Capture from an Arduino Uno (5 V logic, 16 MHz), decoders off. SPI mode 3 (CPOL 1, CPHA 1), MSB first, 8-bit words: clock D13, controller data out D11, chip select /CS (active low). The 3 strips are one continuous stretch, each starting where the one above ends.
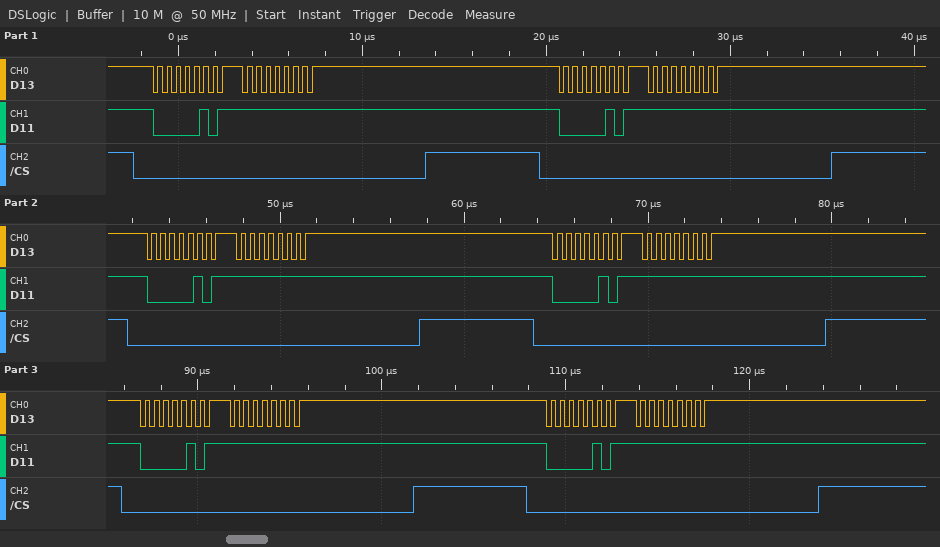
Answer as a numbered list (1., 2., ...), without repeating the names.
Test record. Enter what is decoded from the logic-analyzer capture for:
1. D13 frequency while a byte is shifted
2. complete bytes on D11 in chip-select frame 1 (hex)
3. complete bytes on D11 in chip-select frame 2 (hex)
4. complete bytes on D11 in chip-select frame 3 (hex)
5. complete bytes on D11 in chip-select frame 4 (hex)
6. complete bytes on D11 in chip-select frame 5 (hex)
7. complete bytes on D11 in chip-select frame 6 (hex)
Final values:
1. 2 MHz
2. 0x05 0xFF
3. 0x05 0xFF
4. 0x05 0xFF
5. 0x05 0xFF
6. 0x05 0xFF
7. 0x05 0xFF
